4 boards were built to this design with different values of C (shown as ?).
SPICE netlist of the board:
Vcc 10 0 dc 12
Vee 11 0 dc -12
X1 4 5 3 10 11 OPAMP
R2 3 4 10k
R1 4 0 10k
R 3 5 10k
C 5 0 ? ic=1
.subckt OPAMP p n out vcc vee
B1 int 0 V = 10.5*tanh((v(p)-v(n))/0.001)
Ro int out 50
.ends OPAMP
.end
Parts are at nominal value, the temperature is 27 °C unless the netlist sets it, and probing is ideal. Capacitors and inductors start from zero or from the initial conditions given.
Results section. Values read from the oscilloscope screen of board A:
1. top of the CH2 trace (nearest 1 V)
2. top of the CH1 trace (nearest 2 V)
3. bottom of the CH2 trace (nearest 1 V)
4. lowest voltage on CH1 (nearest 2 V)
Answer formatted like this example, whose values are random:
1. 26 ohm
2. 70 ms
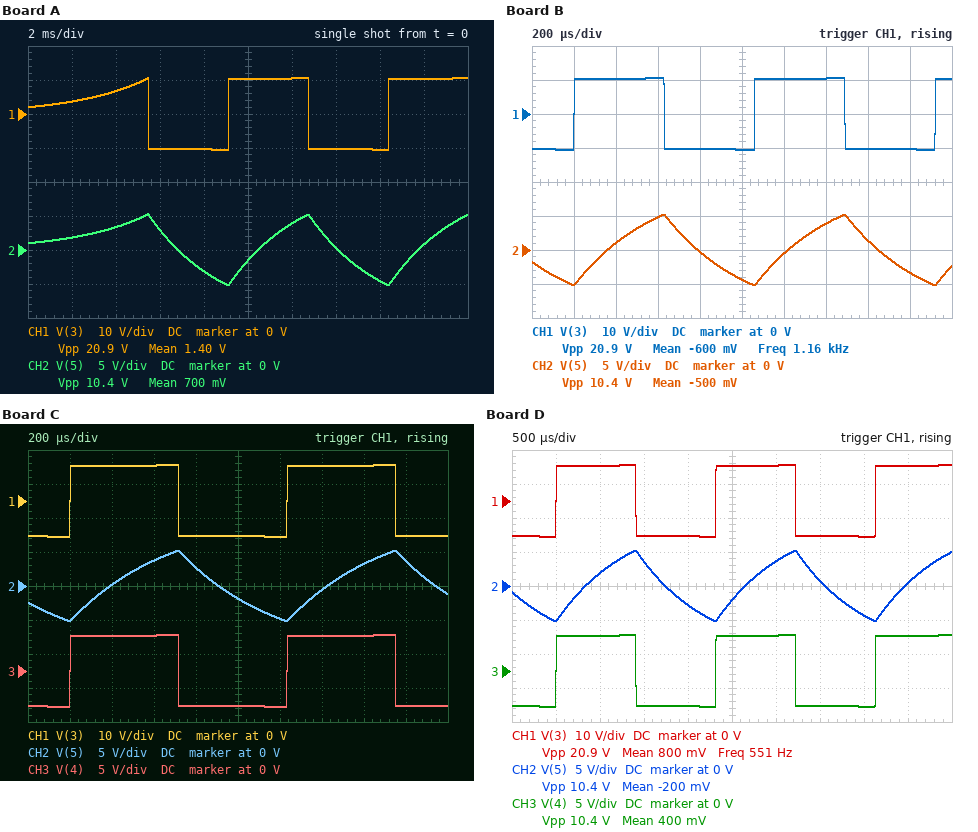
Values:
1. 5 V
2. 10 V
3. -5 V
4. -10 V
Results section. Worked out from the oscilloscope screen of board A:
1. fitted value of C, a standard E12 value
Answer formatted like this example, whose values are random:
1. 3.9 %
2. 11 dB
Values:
1. 330 nF
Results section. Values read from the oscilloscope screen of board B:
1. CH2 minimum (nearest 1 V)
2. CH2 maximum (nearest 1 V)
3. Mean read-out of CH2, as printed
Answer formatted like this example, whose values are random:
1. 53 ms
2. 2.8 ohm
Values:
1. -5 V
2. 5 V
3. -500 mV
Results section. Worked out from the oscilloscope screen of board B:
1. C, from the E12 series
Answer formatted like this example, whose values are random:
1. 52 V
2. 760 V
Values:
1. 39 nF
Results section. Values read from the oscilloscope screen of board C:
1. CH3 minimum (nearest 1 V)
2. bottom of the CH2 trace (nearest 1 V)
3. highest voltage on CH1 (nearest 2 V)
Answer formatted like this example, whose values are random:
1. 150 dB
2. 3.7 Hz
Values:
1. -5 V
2. -5 V
3. 10 V
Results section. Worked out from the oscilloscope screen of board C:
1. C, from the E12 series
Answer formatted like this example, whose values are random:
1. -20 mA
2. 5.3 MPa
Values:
1. 47 nF
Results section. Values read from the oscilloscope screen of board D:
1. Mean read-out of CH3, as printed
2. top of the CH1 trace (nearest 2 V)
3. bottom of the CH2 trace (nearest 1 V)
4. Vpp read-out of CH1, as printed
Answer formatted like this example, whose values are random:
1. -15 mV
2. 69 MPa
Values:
1. 400 mV
2. 10 V
3. -5 V
4. 20.9 V
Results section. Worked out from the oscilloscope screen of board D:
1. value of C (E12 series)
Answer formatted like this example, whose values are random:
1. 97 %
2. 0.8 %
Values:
1. 82 nF
